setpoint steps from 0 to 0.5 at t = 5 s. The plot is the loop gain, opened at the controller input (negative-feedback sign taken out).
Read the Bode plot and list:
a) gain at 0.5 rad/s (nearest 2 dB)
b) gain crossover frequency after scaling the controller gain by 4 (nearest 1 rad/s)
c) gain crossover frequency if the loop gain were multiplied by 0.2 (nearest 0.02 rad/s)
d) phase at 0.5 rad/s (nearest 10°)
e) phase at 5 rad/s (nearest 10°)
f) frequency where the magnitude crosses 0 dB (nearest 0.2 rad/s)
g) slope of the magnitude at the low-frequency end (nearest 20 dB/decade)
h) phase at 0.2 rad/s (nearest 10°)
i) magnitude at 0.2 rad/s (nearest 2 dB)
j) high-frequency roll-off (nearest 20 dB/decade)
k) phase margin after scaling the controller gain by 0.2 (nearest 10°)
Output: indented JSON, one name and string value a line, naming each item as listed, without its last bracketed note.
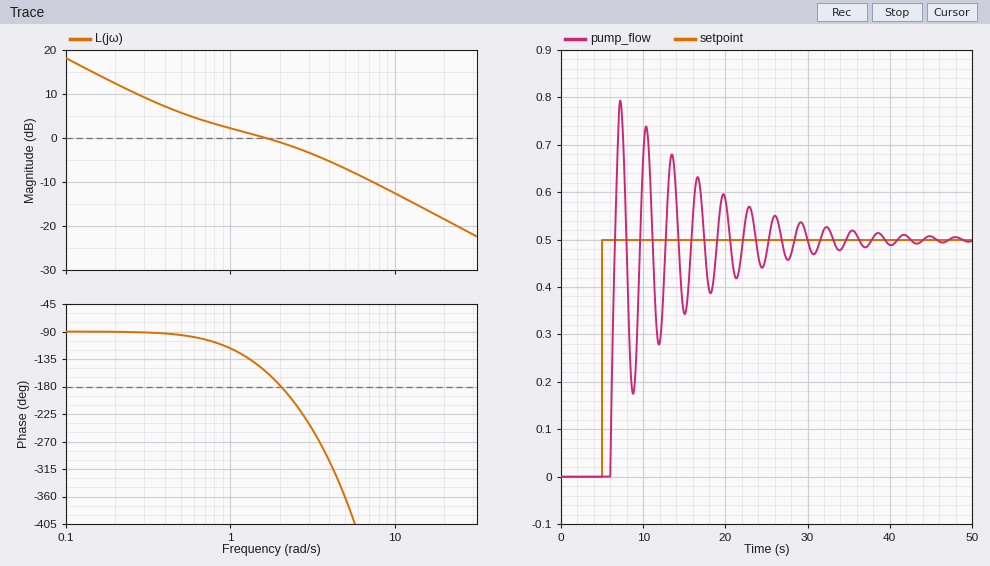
{
  "gain at 0.5 rad/s": "6 dB",
  "gain crossover frequency after scaling the controller gain by 4": "9 rad/s",
  "gain crossover frequency if the loop gain were multiplied by 0.2": "0.16 rad/s",
  "phase at 0.5 rad/s": "-100°",
  "phase at 5 rad/s": "-360°",
  "frequency where the magnitude crosses 0 dB": "1.6 rad/s",
  "slope of the magnitude at the low-frequency end": "-20 dB/decade",
  "phase at 0.2 rad/s": "-90°",
  "magnitude at 0.2 rad/s": "12 dB",
  "high-frequency roll-off": "-20 dB/decade",
  "phase margin after scaling the controller gain by 0.2": "90°"
}
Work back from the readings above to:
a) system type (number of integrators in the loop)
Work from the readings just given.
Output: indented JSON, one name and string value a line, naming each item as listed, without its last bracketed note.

{
  "system type": "1"
}
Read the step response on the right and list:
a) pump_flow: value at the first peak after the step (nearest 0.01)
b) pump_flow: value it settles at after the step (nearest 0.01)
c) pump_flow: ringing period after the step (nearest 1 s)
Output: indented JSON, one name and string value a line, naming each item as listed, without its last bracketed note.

{
  "pump_flow: value at the first peak after the step": "0.79",
  "pump_flow: value it settles at after the step": "0.50",
  "pump_flow: ringing period after the step": "3 s"
}
